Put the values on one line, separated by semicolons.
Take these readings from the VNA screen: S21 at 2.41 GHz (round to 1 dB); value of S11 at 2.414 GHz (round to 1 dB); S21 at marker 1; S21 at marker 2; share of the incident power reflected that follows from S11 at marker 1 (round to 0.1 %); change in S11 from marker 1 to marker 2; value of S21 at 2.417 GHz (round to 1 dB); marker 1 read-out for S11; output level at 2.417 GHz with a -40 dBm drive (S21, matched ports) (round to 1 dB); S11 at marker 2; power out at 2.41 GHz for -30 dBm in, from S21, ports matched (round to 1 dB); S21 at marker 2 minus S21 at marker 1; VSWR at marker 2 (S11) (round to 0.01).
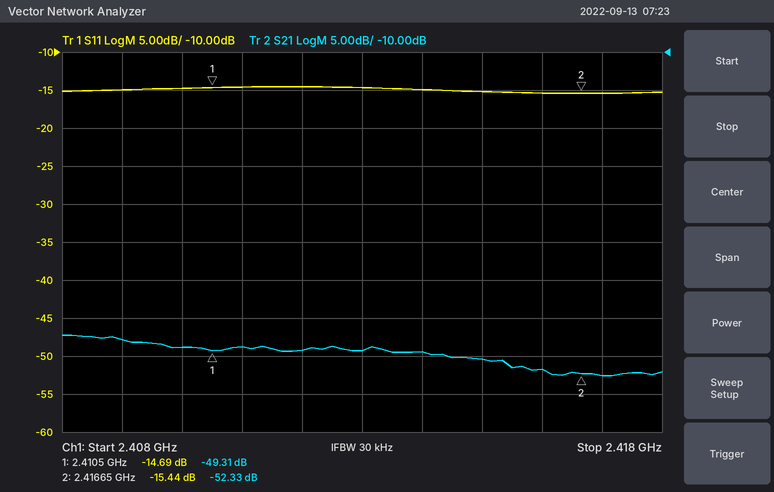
-49 dB; -15 dB; -49.31 dB; -52.33 dB; 3.4 %; -0.75 dB; -53 dB; -14.69 dB; -93 dBm; -15.44 dB; -79 dBm; -3.02 dB; 1.41
